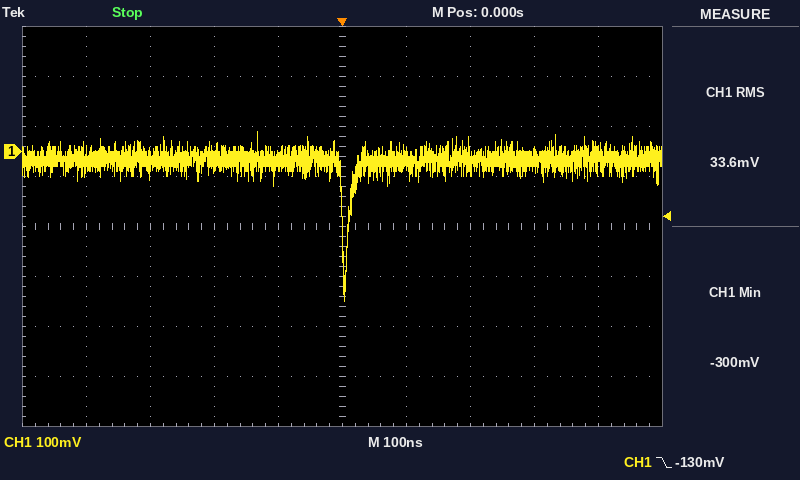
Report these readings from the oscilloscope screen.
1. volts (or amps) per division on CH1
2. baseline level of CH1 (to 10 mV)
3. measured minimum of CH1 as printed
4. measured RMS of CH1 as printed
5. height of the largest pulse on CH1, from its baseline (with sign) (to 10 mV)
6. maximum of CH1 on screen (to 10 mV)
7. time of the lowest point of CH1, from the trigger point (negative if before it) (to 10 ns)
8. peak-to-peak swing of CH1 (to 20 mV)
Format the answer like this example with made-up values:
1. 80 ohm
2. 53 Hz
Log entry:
1. 100 mV
2. -20 mV
3. -300 mV
4. 33.6 mV
5. -280 mV
6. 40 mV
7. 0 ns
8. 340 mV
